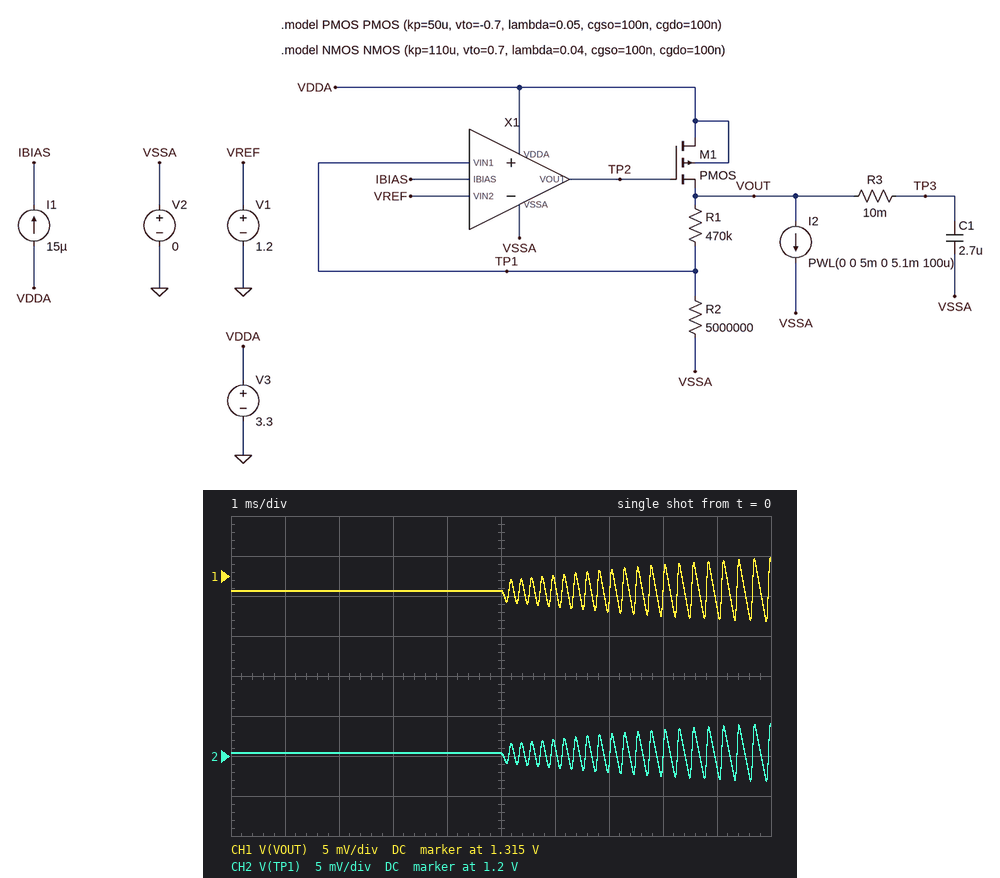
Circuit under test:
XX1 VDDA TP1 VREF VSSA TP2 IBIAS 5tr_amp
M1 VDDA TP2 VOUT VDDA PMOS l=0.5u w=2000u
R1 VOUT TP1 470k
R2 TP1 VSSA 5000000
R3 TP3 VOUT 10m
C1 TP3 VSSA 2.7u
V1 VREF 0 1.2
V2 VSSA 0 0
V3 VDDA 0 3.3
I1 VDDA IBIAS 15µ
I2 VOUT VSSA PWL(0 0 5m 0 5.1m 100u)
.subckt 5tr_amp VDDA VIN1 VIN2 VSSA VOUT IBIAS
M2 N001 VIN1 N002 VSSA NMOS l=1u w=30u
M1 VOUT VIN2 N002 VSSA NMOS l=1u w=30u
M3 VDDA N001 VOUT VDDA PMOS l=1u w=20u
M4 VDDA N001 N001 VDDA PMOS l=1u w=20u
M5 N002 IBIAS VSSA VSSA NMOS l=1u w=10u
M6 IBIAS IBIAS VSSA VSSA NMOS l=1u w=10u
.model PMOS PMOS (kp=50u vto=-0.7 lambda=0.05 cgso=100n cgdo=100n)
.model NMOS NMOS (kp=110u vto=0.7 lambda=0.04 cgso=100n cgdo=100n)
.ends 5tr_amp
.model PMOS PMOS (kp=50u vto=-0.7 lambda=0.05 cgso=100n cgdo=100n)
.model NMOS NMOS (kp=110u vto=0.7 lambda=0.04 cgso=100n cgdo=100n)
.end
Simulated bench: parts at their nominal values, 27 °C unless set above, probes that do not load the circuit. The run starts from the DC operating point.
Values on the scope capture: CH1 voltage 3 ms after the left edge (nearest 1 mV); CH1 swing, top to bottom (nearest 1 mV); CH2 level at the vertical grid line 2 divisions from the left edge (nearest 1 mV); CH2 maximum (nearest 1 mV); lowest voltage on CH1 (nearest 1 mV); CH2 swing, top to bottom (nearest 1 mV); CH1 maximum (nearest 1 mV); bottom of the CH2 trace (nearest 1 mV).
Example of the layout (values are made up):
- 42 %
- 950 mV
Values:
- 1.313 V
- 8 mV
- 1.200 V
- 1.204 V
- 1.309 V
- 7 mV
- 1.317 V
- 1.197 V
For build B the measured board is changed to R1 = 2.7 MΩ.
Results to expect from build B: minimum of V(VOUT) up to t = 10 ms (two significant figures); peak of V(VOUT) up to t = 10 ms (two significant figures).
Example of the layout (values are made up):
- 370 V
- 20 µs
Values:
- 1.8 V
- 1.9 V
